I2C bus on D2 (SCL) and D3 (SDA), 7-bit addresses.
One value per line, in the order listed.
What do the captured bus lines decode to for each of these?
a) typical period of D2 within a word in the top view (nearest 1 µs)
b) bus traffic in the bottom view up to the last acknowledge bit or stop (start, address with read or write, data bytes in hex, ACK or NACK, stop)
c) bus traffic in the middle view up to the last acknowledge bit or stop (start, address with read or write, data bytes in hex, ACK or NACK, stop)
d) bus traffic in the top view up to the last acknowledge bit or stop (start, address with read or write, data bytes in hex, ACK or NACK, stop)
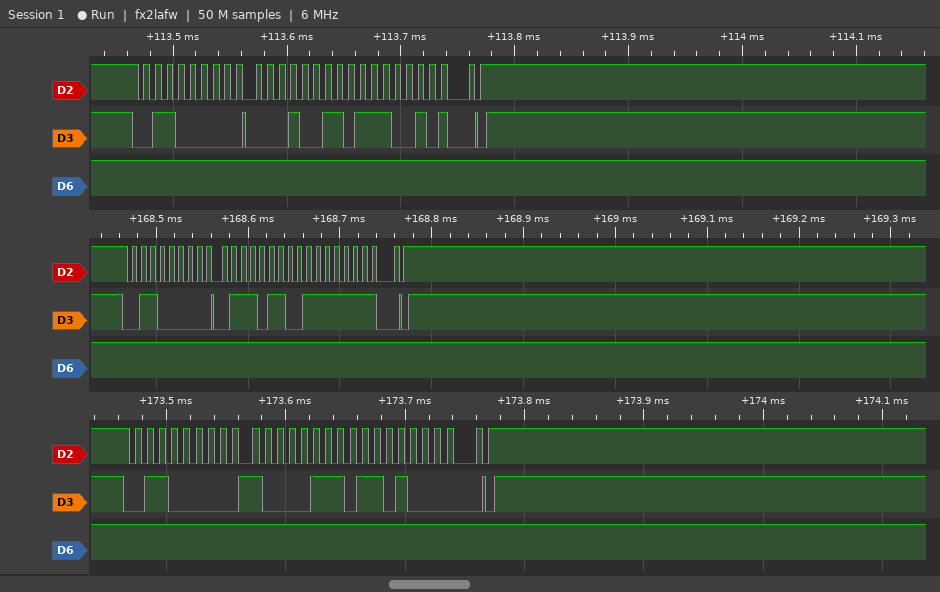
10 µs
start, address 30 write ACK, 87 ACK, D0 ACK, stop
start, address 30 write ACK, 76 ACK, FF ACK, stop
start, address 30 write ACK, 13 ACK, E5 ACK, stop
